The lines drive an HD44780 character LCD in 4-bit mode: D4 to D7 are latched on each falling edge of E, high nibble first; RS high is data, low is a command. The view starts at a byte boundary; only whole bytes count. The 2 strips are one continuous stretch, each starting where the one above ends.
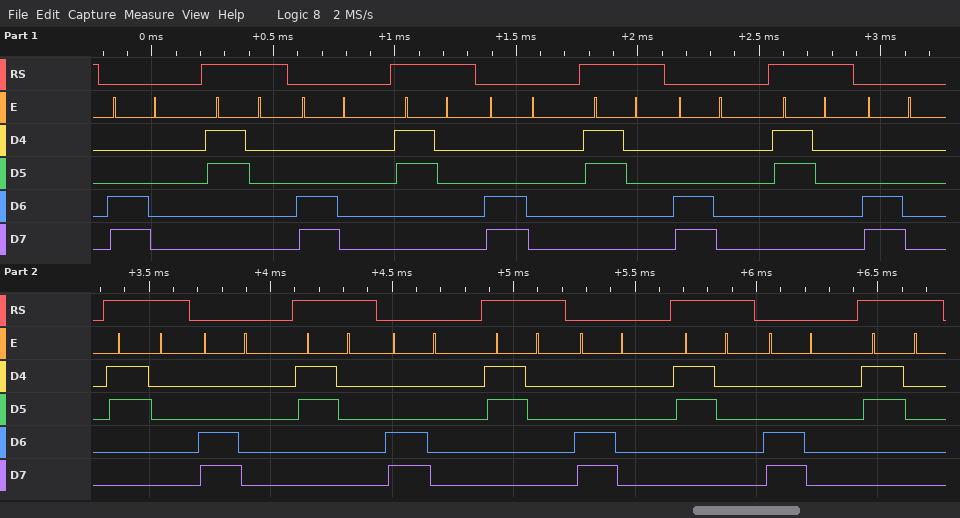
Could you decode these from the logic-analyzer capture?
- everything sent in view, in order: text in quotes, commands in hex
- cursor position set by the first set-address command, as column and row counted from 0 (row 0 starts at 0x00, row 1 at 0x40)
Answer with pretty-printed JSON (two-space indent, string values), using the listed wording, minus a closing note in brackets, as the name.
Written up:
{
  "everything sent in view, in order: text in quotes, commands in hex": "0xC0 \"0\" 0xC0 \"0\" 0xC0 \"0\" 0xC0 \"0\" 0xC0 \"0\" 0xC0 \"0\" 0xC0 \"0\" 0xC0 \"0\" 0xC0 \"0\"",
  "cursor position set by the first set-address command, as column and row counted from 0": "column 0, row 1"
}
